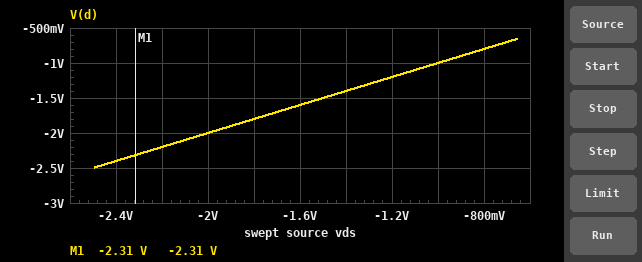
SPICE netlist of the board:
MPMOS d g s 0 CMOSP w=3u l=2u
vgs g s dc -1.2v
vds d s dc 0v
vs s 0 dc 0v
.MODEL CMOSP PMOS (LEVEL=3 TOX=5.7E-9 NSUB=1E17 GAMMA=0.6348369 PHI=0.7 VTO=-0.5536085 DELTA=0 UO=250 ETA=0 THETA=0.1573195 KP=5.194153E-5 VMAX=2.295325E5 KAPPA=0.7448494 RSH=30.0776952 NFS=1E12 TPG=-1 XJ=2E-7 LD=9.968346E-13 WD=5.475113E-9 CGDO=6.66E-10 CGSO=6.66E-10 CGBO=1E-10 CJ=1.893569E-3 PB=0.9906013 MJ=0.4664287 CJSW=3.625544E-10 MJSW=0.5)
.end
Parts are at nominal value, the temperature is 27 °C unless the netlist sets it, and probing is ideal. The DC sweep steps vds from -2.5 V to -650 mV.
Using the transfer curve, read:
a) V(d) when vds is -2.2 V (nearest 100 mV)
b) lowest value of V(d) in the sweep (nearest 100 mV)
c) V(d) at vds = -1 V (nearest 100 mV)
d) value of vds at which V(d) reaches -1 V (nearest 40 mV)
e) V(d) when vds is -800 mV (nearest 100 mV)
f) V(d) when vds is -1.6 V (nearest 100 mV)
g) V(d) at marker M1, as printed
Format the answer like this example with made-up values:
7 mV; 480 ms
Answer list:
-2.2 V; -2.5 V; -1.0 V; -1.00 V; -800 mV; -1.6 V; -2.31 V
